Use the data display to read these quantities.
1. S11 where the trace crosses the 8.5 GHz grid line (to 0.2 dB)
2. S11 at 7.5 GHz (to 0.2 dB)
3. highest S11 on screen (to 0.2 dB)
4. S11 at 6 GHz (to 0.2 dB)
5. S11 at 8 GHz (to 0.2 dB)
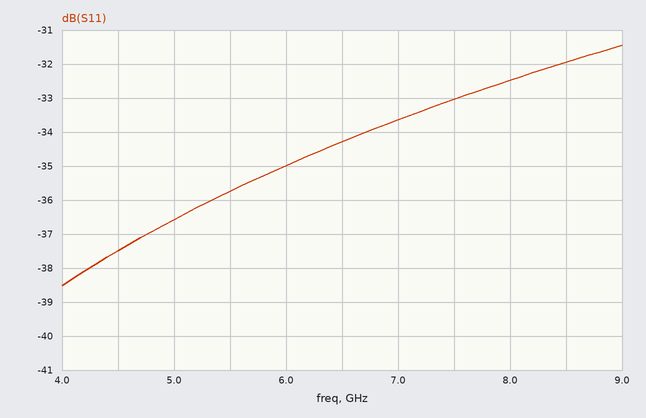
-32.0 dB
-33.0 dB
-31.4 dB
-35.0 dB
-32.4 dB
